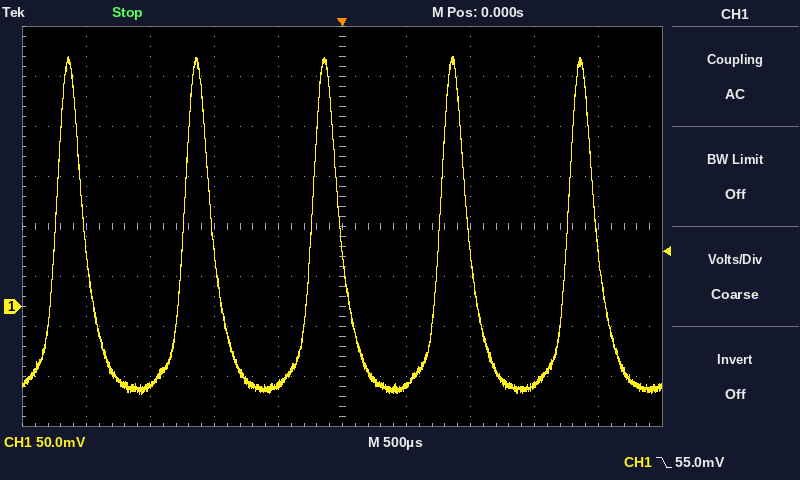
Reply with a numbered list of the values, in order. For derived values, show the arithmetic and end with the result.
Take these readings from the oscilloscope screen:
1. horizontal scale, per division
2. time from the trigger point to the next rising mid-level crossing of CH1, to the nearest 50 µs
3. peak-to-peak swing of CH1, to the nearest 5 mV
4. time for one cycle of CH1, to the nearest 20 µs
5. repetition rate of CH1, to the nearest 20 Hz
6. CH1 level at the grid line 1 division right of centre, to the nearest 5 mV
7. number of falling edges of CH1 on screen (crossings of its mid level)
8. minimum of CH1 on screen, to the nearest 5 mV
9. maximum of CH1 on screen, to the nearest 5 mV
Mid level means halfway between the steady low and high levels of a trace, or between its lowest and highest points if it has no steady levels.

1. 500 µs
2. 750 µs
3. 250 mV − (-90 mV) = 340 mV
4. 1.00 ms
5. 1 / 1.00 ms ≈ 1.00 kHz
6. -80 mV
7. 5
8. -90 mV
9. 250 mV
